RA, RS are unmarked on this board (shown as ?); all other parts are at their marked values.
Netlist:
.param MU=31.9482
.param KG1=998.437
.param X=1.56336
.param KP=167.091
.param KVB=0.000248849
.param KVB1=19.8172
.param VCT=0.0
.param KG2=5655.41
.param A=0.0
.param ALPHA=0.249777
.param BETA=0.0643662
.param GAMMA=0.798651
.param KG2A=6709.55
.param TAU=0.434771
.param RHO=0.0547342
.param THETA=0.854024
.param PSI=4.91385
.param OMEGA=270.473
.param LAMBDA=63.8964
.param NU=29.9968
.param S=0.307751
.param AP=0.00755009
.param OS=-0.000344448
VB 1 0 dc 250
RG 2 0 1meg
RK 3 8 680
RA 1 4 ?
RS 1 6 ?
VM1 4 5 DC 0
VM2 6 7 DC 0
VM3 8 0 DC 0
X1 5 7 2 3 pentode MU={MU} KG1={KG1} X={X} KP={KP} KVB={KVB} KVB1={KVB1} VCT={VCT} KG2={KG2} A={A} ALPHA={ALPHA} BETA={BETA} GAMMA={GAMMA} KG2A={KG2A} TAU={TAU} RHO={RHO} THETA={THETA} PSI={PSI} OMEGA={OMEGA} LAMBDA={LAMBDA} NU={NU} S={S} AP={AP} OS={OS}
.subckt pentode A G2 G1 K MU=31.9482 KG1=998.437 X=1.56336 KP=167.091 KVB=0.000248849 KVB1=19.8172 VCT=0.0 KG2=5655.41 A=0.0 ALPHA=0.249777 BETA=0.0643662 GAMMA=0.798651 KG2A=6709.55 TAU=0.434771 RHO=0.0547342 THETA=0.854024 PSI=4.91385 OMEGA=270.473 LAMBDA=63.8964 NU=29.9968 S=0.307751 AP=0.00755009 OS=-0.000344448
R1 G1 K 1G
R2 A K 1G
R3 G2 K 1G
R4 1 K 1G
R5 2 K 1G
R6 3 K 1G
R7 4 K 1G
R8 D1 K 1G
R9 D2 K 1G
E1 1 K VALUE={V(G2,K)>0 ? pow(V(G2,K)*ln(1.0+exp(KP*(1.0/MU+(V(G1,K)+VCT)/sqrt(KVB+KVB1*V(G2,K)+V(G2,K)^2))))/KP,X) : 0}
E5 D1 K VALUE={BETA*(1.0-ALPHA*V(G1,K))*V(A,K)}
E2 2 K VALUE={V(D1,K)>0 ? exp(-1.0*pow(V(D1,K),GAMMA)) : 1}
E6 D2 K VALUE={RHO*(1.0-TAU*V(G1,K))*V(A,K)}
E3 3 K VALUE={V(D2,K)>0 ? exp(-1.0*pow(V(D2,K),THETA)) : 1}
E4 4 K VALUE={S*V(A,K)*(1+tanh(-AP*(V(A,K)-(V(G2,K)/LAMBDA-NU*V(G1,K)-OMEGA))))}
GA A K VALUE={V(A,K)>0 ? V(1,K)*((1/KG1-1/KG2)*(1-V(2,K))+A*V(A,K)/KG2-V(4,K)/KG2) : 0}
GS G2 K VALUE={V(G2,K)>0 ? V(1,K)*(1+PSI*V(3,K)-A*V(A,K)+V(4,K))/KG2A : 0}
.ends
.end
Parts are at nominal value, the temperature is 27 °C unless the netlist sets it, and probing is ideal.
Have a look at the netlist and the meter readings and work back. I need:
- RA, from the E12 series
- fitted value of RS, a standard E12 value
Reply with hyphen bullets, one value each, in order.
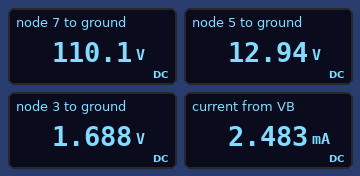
- 180 kΩ
- 120 kΩ
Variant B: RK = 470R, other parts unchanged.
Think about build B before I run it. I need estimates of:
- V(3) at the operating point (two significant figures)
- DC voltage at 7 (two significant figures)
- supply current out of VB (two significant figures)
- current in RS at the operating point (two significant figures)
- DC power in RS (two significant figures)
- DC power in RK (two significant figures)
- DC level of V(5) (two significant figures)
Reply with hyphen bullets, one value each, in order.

- 1.2 V
- 97 V
- 2.6 mA
- 1.3 mA
- 190 mW
- 3.2 mW
- 12 V
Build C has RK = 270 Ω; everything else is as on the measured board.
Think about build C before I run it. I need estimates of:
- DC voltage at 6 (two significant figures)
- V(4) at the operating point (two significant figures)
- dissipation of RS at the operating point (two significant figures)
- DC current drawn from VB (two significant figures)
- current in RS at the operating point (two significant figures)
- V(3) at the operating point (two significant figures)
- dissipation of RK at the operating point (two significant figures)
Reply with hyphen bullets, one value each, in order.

- 84 V
- 12 V
- 230 mW
- 2.7 mA
- 1.4 mA
- 730 mV
- 2.0 mW
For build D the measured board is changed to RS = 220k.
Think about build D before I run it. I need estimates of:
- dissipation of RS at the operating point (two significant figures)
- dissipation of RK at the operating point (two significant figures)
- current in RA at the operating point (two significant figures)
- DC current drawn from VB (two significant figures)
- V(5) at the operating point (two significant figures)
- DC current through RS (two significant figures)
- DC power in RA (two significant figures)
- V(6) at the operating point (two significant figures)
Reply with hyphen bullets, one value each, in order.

- 110 mW
- 2.7 mW
- 1.3 mA
- 2.0 mA
- 21 V
- 720 µA
- 290 mW
- 91 V
